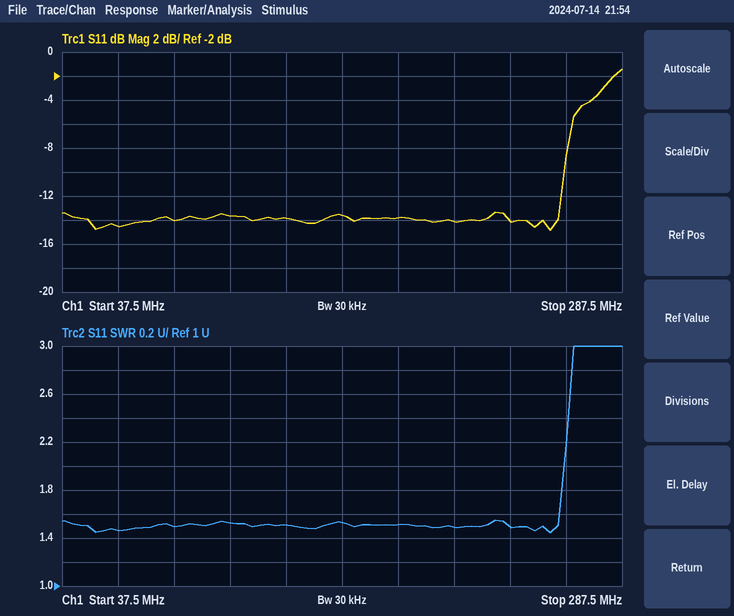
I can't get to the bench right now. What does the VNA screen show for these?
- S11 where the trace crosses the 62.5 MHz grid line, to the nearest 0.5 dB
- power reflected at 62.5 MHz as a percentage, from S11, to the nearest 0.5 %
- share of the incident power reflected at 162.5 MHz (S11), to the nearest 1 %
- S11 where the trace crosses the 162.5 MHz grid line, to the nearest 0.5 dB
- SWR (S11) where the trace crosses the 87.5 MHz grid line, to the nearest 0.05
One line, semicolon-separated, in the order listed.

-14.5 dB; 3.5 %; 4 %; -13.5 dB; 1.50
